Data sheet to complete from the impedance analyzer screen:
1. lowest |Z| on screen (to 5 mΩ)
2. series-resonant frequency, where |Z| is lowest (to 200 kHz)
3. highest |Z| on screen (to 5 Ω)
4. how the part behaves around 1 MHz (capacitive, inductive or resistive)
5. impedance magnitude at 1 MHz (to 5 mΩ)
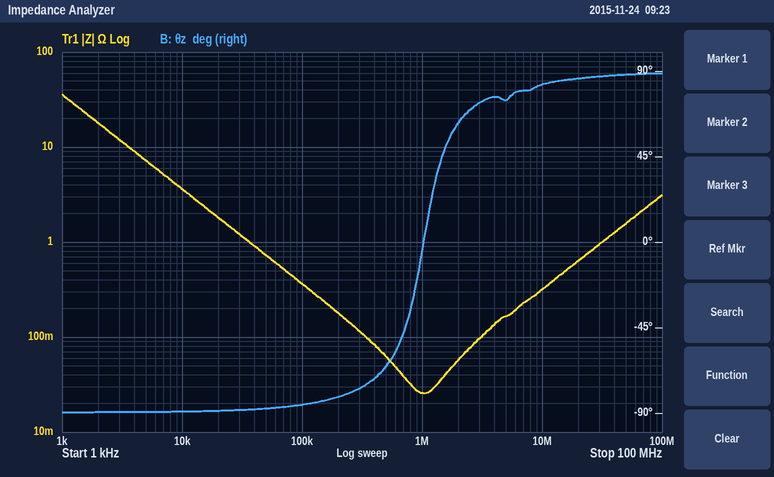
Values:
25 mΩ
1.0 MHz
35 Ω
resistive
25 mΩ
